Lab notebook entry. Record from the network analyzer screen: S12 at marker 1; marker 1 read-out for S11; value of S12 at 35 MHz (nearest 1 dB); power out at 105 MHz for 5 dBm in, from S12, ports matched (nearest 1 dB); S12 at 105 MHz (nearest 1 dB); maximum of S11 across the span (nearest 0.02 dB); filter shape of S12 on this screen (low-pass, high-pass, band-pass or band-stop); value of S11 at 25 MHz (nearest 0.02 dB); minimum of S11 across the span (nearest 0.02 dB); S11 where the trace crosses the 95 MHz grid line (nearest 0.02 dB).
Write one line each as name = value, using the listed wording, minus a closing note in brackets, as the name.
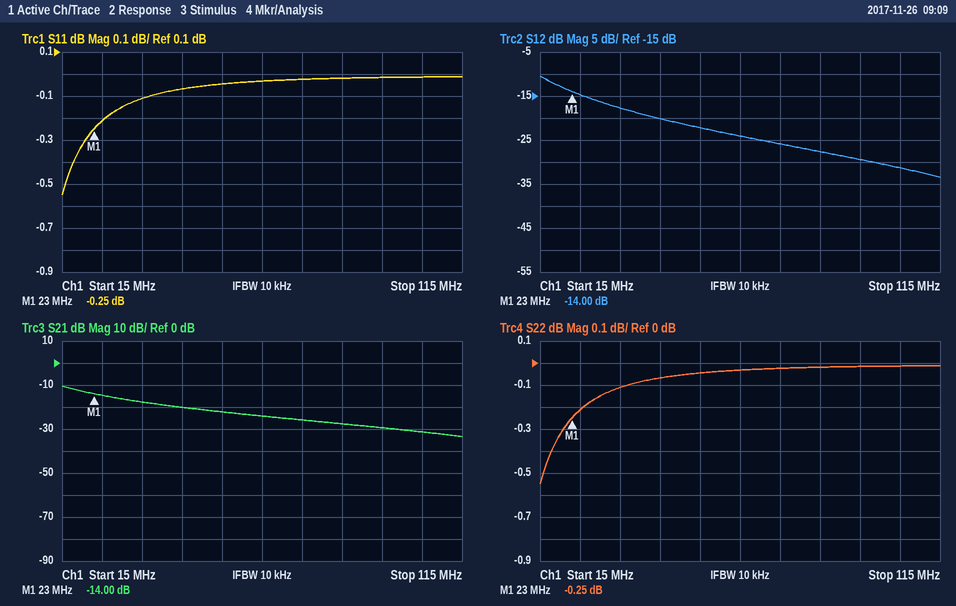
S12 at marker 1 = -14.00 dB
marker 1 read-out for S11 = -0.25 dB
value of S12 at 35 MHz = -18 dB
power out at 105 MHz for 5 dBm in, from S12, ports matched = -26 dBm
S12 at 105 MHz = -31 dB
maximum of S11 across the span = -0.02 dB
filter shape of S12 on this screen = low-pass
value of S11 at 25 MHz = -0.22 dB
minimum of S11 across the span = -0.54 dB
S11 where the trace crosses the 95 MHz grid line = -0.02 dB
